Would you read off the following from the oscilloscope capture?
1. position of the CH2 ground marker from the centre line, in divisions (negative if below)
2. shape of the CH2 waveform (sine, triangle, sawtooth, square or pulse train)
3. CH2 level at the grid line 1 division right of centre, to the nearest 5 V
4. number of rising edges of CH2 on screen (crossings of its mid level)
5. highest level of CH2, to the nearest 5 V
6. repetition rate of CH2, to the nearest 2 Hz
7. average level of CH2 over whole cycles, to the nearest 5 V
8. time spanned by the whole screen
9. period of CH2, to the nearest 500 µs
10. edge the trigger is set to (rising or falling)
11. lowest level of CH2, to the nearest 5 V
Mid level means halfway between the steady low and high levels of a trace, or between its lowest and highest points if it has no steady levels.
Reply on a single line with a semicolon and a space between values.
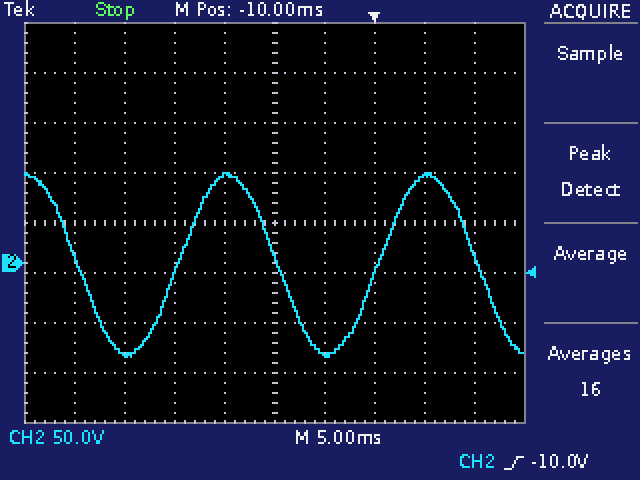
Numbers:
-0.8 div; sine; -90 V; 2; 90 V; 50 Hz; 0 V; 50 ms; 20.0 ms; rising; -95 V
